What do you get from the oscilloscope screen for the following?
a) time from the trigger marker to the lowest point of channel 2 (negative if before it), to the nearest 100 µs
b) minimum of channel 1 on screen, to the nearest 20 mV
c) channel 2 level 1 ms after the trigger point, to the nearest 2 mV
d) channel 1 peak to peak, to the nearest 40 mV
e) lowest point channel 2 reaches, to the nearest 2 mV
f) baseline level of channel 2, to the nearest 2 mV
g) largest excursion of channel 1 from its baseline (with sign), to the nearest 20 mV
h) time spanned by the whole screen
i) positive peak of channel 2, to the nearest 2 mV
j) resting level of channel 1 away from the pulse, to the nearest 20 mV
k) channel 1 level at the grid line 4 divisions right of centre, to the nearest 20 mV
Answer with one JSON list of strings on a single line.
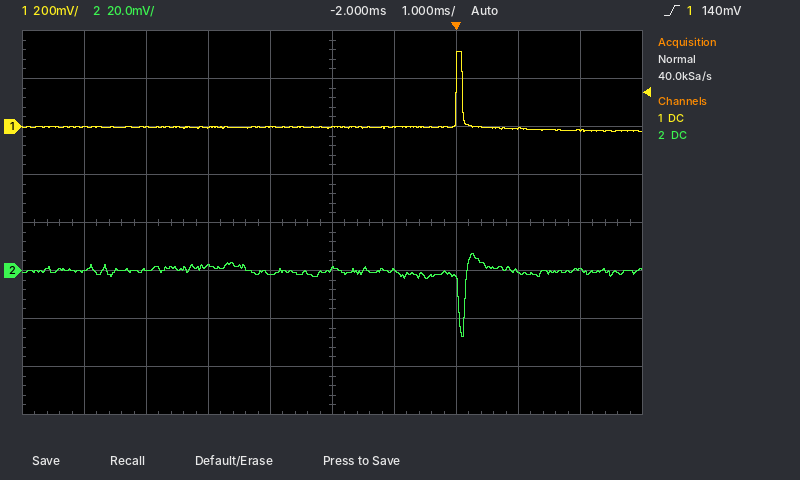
["+100 µs", "-20 mV", "0 mV", "320 mV", "-28 mV", "0 mV", "+320 mV", "10 ms", "8 mV", "0 mV", "-20 mV"]
